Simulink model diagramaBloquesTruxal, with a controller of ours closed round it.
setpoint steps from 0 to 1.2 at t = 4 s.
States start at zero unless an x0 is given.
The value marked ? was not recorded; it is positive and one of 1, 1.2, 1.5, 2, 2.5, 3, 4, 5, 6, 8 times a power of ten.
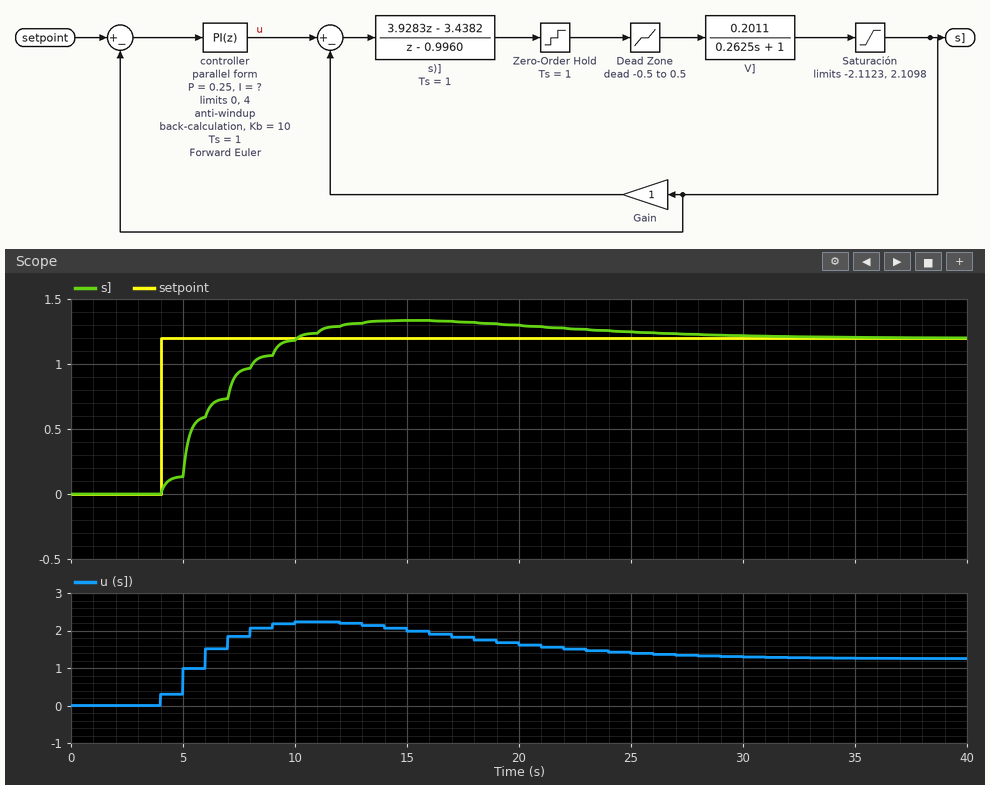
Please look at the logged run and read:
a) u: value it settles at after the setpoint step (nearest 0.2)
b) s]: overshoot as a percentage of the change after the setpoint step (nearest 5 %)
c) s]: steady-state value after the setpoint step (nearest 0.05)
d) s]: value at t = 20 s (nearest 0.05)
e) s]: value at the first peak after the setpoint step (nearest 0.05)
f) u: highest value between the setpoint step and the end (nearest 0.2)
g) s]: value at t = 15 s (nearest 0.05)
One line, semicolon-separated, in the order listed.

1.2; 10 %; 1.20; 1.30; 1.35; 2.2; 1.35
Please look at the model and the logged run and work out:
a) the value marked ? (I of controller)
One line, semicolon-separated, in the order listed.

0.6
